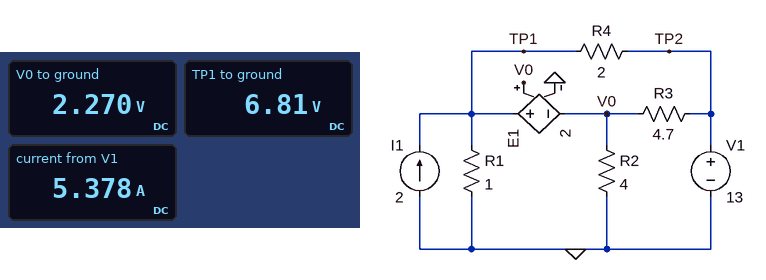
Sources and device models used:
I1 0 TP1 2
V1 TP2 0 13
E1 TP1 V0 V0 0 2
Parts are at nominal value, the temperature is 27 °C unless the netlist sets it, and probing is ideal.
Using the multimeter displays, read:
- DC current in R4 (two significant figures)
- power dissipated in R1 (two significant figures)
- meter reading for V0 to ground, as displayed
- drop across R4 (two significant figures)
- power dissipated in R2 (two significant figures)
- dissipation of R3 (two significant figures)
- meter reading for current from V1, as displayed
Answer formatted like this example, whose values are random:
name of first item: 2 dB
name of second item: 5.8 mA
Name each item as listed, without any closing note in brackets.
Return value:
DC current in R4: 3.1 A
power dissipated in R1: 46 W
meter reading for V0 to ground, as displayed: 2.270 V
drop across R4: 6.2 V
power dissipated in R2: 1.3 W
dissipation of R3: 24 W
meter reading for current from V1, as displayed: 5.378 A
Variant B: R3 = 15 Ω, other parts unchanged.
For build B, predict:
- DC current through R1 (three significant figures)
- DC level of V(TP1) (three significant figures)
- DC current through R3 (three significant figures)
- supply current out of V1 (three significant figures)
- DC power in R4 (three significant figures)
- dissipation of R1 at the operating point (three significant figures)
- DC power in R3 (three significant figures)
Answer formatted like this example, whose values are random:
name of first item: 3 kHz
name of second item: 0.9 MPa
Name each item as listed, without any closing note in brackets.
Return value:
DC current through R1: 5.83 A
DC level of V(TP1): 5.83 V
DC current through R3: 737 mA
supply current out of V1: 4.32 A
DC power in R4: 25.7 W
dissipation of R1 at the operating point: 34.0 W
DC power in R3: 8.15 W
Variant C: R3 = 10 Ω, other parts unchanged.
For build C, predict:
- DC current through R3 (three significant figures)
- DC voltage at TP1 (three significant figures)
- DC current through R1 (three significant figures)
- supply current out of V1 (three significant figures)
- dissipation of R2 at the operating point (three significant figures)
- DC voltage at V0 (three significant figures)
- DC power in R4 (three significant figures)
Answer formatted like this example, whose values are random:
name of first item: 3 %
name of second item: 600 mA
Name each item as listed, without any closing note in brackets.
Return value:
DC current through R3: 1.10 A
DC voltage at TP1: 6.06 V
DC current through R1: 6.06 A
supply current out of V1: 4.57 A
dissipation of R2 at the operating point: 1.02 W
DC voltage at V0: 2.02 V
DC power in R4: 24.1 W
